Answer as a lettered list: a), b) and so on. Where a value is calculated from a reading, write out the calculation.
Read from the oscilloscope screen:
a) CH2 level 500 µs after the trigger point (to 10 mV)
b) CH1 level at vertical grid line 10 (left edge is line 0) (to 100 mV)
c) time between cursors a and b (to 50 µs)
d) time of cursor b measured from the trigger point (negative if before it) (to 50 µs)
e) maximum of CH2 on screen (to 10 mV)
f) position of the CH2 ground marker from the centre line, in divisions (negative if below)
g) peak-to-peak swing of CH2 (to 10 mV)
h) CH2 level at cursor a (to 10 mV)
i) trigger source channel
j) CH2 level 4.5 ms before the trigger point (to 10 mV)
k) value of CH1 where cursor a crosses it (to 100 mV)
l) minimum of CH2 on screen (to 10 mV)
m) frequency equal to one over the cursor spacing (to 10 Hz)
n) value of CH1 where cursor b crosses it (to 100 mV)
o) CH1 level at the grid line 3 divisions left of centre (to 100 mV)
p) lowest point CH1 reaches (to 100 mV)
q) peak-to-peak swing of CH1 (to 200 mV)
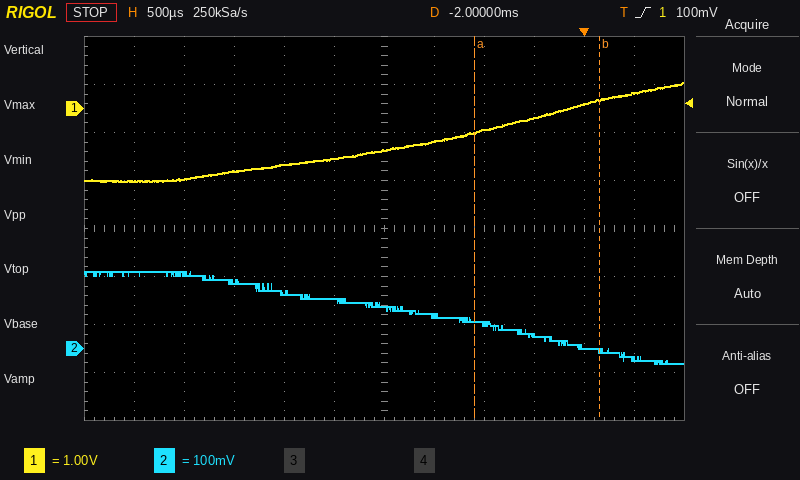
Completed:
a) -20 mV
b) 100 mV
c) 1.25 ms
d) +150 µs
e) 160 mV
f) -2.5 div
g) 160 mV − (-30 mV) = 190 mV
h) 60 mV
i) CH1
j) 160 mV
k) -500 mV
l) -30 mV
m) 1 / 1.25 ms ≈ 800 Hz
n) 200 mV
o) -1.3 V
p) -1.5 V
q) 2.0 V
